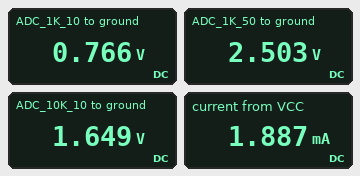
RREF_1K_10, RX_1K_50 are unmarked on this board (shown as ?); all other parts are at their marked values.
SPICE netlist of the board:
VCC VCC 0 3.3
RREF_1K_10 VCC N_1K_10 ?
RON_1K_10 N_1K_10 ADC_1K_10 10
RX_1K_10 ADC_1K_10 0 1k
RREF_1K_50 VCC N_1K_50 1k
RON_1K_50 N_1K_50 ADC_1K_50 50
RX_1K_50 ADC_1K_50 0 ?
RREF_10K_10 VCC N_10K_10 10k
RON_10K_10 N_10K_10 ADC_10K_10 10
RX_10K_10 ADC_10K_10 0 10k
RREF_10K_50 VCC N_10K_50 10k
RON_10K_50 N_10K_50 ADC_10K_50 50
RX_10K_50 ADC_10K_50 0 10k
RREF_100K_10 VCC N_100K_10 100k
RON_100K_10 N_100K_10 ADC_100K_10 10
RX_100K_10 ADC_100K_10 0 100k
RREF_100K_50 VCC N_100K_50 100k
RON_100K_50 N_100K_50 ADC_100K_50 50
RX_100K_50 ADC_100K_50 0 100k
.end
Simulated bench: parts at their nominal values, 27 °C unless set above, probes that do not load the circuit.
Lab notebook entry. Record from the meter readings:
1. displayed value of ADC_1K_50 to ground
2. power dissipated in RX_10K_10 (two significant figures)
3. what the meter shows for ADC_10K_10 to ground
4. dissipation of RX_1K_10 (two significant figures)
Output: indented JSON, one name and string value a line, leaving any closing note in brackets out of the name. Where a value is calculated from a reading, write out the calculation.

{
  "displayed value of ADC_1K_50 to ground": "2.503 V",
  "power dissipated in RX_10K_10": "(1.649 V)^2 / 10 kΩ = 270 µW",
  "what the meter shows for ADC_10K_10 to ground": "1.649 V",
  "dissipation of RX_1K_10": "(766 mV)^2 / 1 kΩ = 590 µW"
}
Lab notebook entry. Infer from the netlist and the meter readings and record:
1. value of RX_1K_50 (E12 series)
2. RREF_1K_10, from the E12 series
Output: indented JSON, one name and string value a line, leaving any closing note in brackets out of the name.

{
  "value of RX_1K_50": "3.3 kΩ",
  "RREF_1K_10, from the E12 series": "3.3 kΩ"
}
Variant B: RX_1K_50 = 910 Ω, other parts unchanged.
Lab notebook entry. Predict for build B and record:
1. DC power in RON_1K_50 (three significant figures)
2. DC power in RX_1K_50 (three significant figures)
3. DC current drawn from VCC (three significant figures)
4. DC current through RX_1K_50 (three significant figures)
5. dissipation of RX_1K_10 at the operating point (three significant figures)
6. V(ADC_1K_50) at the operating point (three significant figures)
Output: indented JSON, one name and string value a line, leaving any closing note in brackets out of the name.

{
  "DC power in RON_1K_50": "142 µW",
  "DC power in RX_1K_50": "2.58 mW",
  "DC current drawn from VCC": "2.81 mA",
  "DC current through RX_1K_50": "1.68 mA",
  "dissipation of RX_1K_10 at the operating point": "586 µW",
  "V(ADC_1K_50) at the operating point": "1.53 V"
}
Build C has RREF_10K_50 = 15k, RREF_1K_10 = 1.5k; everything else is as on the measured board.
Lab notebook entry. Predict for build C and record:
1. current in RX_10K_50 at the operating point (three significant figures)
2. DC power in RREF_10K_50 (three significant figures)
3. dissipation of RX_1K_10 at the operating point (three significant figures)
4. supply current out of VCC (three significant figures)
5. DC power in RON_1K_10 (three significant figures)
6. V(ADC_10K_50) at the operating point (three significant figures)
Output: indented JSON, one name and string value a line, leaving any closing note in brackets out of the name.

{
  "current in RX_10K_50 at the operating point": "132 µA",
  "DC power in RREF_10K_50": "260 µW",
  "dissipation of RX_1K_10 at the operating point": "1.73 mW",
  "supply current out of VCC": "2.40 mA",
  "DC power in RON_1K_10": "17.3 µW",
  "V(ADC_10K_50) at the operating point": "1.32 V"
}
